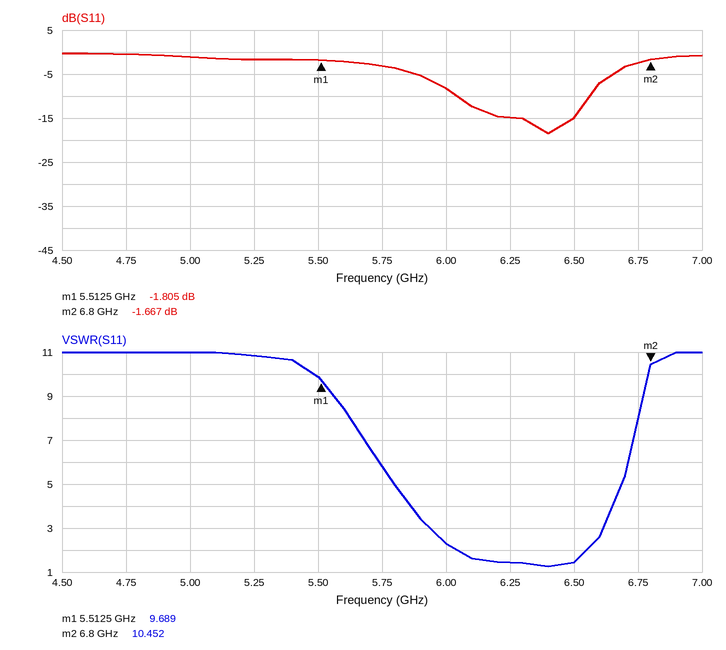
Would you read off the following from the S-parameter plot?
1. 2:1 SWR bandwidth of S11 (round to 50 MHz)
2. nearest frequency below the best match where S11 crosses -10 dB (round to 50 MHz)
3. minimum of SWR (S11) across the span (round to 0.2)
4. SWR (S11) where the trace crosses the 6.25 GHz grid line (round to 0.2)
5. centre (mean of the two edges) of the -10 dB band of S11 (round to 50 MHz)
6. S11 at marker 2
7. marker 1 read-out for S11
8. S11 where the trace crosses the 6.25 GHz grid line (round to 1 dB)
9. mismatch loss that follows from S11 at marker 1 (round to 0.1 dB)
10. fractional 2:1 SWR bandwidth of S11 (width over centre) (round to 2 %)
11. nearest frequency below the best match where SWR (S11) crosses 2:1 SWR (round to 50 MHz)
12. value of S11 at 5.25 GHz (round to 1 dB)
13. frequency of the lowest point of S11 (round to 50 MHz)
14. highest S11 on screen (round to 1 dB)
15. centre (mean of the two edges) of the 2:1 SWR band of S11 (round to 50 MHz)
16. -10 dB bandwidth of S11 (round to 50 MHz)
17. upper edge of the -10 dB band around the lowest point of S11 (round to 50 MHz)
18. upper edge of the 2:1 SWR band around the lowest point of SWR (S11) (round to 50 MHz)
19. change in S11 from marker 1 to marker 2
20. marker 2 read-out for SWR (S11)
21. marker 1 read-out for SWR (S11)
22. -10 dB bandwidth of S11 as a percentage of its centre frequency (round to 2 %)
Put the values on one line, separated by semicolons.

500 MHz; 6.05 GHz; 1.2; 1.4; 6.30 GHz; -1.667 dB; -1.805 dB; -15 dB; 4.7 dB; 8 %; 6.05 GHz; -2 dB; 6.40 GHz; 0 dB; 6.30 GHz; 500 MHz; 6.55 GHz; 6.55 GHz; 0.138 dB; 10.452; 9.689; 8 %
